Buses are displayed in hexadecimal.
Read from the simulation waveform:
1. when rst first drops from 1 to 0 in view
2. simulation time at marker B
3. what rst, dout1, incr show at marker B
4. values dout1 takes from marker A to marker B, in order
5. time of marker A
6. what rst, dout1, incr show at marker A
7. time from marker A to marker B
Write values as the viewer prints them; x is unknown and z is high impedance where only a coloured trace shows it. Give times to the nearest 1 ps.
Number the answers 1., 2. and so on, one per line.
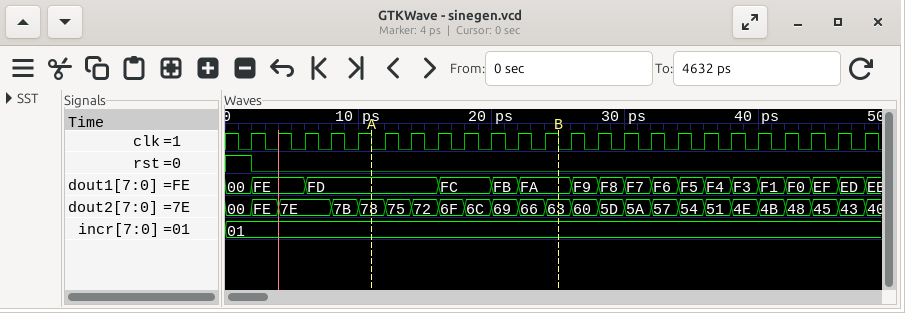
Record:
1. 2 ps
2. 25 ps
3. rst=0, dout1=FA, incr=01
4. FD, FC, FB, FA
5. 11 ps
6. rst=0, dout1=FD, incr=01
7. 14 ps
